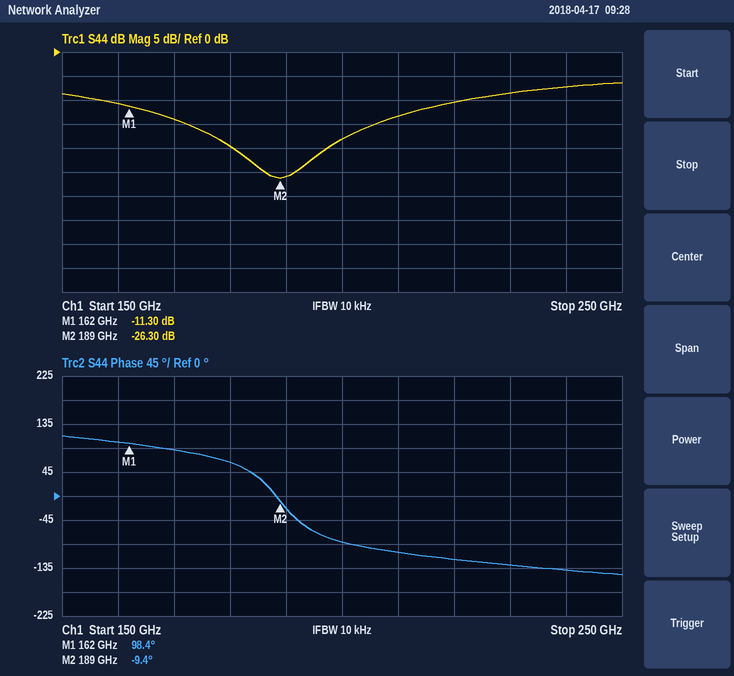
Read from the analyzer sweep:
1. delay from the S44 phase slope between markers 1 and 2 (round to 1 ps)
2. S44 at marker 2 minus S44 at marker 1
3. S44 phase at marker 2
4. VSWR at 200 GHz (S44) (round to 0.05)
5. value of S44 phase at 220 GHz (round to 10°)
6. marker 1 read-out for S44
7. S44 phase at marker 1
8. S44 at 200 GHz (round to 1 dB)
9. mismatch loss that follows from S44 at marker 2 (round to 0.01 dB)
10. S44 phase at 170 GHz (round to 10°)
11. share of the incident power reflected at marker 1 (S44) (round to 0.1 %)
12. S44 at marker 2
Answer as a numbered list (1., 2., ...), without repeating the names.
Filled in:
1. 11 ps
2. -15.00 dB
3. -9.4°
4. 1.30
5. -120°
6. -11.30 dB
7. 98.4°
8. -18 dB
9. 0.01 dB
10. 90°
11. 7.4 %
12. -26.30 dB
